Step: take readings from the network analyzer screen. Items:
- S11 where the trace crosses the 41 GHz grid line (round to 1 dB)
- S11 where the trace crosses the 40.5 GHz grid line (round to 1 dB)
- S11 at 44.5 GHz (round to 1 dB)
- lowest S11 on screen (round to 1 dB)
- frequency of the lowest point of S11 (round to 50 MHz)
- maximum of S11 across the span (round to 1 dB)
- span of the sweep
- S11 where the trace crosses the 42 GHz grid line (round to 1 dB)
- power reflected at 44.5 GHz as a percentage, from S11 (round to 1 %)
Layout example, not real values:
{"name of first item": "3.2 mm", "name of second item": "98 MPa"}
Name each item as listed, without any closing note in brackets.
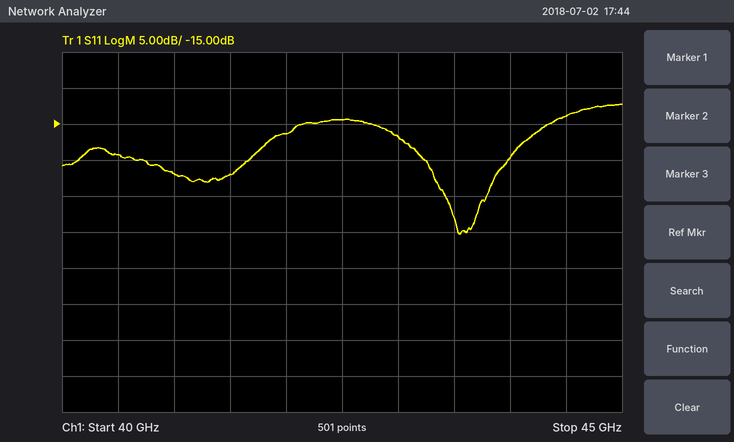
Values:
{"S11 where the trace crosses the 41 GHz grid line": "-22 dB", "S11 where the trace crosses the 40.5 GHz grid line": "-19 dB", "S11 at 44.5 GHz": "-14 dB", "lowest S11 on screen": "-30 dB", "frequency of the lowest point of S11": "43.55 GHz", "maximum of S11 across the span": "-12 dB", "span of the sweep": "5 GHz", "S11 where the trace crosses the 42 GHz grid line": "-16 dB", "power reflected at 44.5 GHz as a percentage, from S11": "4 %"}
